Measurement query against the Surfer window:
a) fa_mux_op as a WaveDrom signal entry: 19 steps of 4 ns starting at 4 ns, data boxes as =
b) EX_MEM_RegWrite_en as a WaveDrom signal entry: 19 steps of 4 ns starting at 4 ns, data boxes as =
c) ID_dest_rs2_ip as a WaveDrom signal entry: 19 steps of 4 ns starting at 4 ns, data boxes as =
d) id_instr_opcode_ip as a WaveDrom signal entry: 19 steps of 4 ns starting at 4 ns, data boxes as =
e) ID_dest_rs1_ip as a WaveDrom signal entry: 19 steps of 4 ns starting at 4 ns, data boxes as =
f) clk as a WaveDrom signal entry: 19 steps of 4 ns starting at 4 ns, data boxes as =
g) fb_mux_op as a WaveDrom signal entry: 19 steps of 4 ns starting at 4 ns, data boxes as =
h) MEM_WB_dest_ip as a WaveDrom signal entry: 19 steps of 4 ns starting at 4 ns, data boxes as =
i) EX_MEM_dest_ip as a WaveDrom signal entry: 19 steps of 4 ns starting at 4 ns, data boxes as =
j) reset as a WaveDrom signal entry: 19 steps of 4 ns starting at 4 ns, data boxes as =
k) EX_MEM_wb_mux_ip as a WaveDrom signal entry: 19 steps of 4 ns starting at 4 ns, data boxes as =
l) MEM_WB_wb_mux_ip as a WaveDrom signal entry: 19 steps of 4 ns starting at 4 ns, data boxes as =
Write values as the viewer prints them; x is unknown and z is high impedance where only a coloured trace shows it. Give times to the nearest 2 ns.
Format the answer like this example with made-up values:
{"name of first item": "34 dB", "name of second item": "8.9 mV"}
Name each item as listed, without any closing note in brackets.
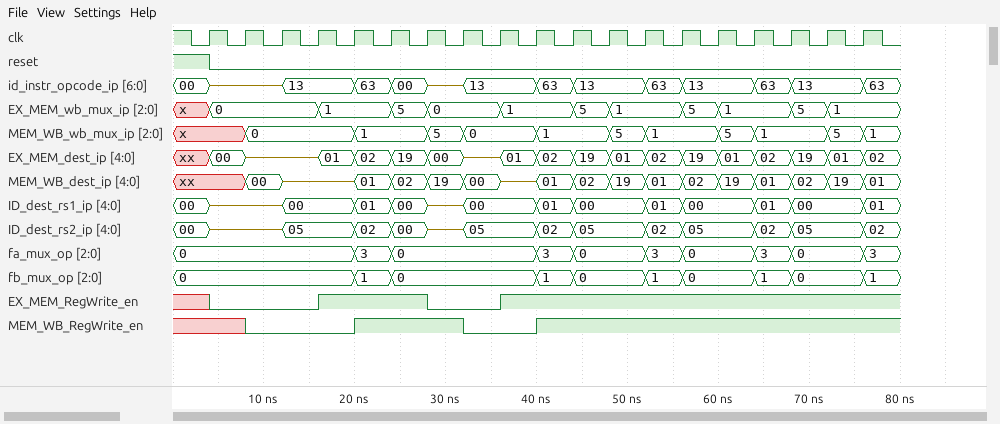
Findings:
{"fa_mux_op as a WaveDrom signal entry: 19 steps of 4 ns starting at 4 ns, data boxes as =": "{name: 'fa_mux_op', wave: '=...==...==.==.==.=', data: '0 3 0 3 0 3 0 3 0 3'}", "EX_MEM_RegWrite_en as a WaveDrom signal entry: 19 steps of 4 ns starting at 4 ns, data boxes as =": "{name: 'EX_MEM_RegWrite_en', wave: '0..1..0.1..........'}", "ID_dest_rs2_ip as a WaveDrom signal entry: 19 steps of 4 ns starting at 4 ns, data boxes as =": "{name: 'ID_dest_rs2_ip', wave: 'z.=.==z=.==.==.==.=', data: '05 02 00 05 02 05 02 05 02 05 02'}", "id_instr_opcode_ip as a WaveDrom signal entry: 19 steps of 4 ns starting at 4 ns, data boxes as =": "{name: 'id_instr_opcode_ip', wave: 'z.=.==z=.==.==.==.=', data: '13 63 00 13 63 13 63 13 63 13 63'}", "ID_dest_rs1_ip as a WaveDrom signal entry: 19 steps of 4 ns starting at 4 ns, data boxes as =": "{name: 'ID_dest_rs1_ip', wave: 'z.=.==z=.==.==.==.=', data: '00 01 00 00 01 00 01 00 01 00 01'}", "clk as a WaveDrom signal entry: 19 steps of 4 ns starting at 4 ns, data boxes as =": "{name: 'clk', wave: 'p..................'}", "fb_mux_op as a WaveDrom signal entry: 19 steps of 4 ns starting at 4 ns, data boxes as =": "{name: 'fb_mux_op', wave: '=...==...==.==.==.=', data: '0 1 0 1 0 1 0 1 0 1'}", "MEM_WB_dest_ip as a WaveDrom signal entry: 19 steps of 4 ns starting at 4 ns, data boxes as =": "{name: 'MEM_WB_dest_ip', wave: 'x=z.====z==========', data: '00 01 02 19 00 01 02 19 01 02 19 01 02 19 01'}", "EX_MEM_dest_ip as a WaveDrom signal entry: 19 steps of 4 ns starting at 4 ns, data boxes as =": "{name: 'EX_MEM_dest_ip', wave: '=z.====z===========', data: '00 01 02 19 00 01 02 19 01 02 19 01 02 19 01 02'}", "reset as a WaveDrom signal entry: 19 steps of 4 ns starting at 4 ns, data boxes as =": "{name: 'reset', wave: '0..................'}", "EX_MEM_wb_mux_ip as a WaveDrom signal entry: 19 steps of 4 ns starting at 4 ns, data boxes as =": "{name: 'EX_MEM_wb_mux_ip', wave: '=..=.==.=.==.==.==.', data: '0 1 5 0 1 5 1 5 1 5 1'}", "MEM_WB_wb_mux_ip as a WaveDrom signal entry: 19 steps of 4 ns starting at 4 ns, data boxes as =": "{name: 'MEM_WB_wb_mux_ip', wave: 'x=..=.==.=.==.==.==', data: '0 1 5 0 1 5 1 5 1 5 1'}"}
